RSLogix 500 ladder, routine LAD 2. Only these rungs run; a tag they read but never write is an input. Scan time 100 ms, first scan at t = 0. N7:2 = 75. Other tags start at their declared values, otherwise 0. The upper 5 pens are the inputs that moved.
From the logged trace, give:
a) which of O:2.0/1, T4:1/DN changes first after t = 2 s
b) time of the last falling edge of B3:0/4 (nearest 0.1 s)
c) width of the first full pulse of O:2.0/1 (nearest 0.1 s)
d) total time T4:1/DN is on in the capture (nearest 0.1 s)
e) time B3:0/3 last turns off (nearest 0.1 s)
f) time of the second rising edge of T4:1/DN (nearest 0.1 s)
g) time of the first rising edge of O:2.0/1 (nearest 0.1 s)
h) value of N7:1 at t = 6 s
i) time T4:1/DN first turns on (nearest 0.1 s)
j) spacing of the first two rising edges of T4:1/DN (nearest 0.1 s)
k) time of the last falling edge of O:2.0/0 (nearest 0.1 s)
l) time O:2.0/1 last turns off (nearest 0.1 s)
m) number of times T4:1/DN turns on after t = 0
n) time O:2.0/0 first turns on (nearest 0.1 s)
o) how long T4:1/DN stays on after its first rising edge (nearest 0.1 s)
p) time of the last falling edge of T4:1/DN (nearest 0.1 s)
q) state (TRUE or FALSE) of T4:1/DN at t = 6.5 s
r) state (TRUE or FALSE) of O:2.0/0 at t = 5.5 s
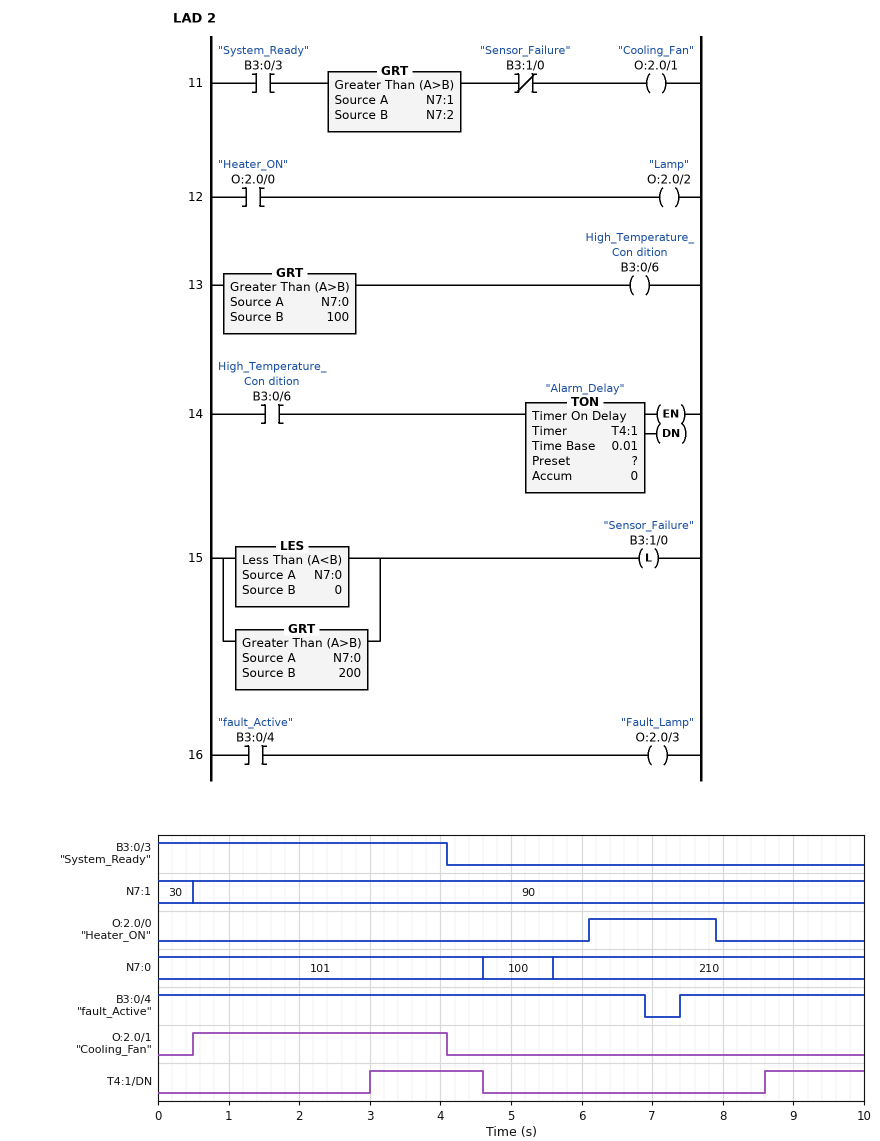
T4:1/DN
6.9 s
3.6 s
3.0 s
4.1 s
8.6 s
0.5 s
90
3.0 s
5.6 s
7.9 s
4.1 s
2
6.1 s
1.6 s
4.6 s
FALSE
FALSE
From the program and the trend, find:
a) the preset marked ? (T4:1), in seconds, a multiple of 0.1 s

3.0 s
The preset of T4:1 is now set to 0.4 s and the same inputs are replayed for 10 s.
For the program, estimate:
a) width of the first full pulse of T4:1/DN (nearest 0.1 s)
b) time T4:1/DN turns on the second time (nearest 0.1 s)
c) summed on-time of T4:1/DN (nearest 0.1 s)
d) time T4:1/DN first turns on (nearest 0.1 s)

4.2 s
6.0 s
8.2 s
0.4 s
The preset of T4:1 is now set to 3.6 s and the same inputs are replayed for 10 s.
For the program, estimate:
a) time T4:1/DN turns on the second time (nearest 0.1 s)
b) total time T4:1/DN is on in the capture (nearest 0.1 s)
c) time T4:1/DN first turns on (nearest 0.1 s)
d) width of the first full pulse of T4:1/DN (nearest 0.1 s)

9.2 s
1.8 s
3.6 s
1.0 s
